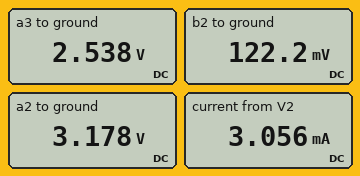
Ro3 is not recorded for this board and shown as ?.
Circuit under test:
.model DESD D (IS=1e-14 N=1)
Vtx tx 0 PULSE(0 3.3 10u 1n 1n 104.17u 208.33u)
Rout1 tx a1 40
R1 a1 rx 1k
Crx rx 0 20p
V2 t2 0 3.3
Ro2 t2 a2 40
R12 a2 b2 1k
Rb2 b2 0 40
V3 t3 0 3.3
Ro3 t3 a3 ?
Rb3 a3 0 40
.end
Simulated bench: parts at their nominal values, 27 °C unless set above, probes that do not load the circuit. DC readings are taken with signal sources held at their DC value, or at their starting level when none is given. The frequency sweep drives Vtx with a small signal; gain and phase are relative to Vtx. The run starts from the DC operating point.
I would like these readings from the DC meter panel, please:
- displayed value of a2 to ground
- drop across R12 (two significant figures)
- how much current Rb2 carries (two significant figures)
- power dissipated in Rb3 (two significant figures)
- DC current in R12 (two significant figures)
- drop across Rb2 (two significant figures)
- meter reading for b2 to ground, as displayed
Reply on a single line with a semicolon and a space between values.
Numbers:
3.178 V; 3.1 V; 3.1 mA; 160 mW; 3.1 mA; 120 mV; 122.2 mV
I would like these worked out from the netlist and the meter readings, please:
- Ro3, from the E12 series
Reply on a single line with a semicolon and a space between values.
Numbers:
12 Ω
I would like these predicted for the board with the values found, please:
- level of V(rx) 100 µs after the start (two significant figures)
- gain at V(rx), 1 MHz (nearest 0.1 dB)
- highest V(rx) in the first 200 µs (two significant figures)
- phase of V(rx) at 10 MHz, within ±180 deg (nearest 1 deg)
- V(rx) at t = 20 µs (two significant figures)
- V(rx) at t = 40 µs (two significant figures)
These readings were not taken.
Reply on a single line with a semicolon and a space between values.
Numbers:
3.3 V; -0.1 dB; 3.3 V; -53 deg; 3.3 V; 3.3 V
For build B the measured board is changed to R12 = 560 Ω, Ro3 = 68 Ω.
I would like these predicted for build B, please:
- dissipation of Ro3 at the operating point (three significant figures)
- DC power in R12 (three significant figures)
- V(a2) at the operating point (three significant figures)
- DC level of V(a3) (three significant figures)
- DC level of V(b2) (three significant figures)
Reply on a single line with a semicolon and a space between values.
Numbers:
63.5 mW; 14.9 mW; 3.09 V; 1.22 V; 206 mV
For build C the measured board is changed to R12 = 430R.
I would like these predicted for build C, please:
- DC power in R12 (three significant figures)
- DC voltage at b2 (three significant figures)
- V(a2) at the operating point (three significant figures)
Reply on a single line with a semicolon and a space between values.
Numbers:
18.0 mW; 259 mV; 3.04 V
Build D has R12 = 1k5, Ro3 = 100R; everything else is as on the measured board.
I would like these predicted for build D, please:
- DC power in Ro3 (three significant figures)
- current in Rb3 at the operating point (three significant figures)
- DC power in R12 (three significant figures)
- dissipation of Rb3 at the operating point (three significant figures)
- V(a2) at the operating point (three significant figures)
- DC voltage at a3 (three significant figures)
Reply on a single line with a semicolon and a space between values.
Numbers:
55.6 mW; 23.6 mA; 6.54 mW; 22.2 mW; 3.22 V; 943 mV
